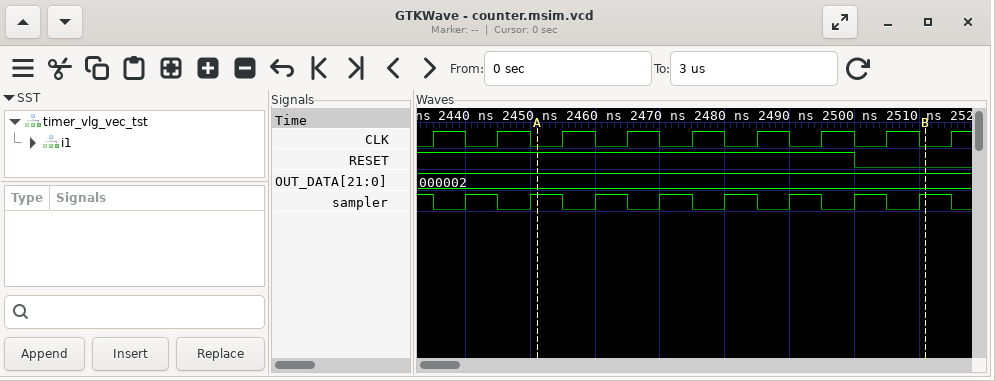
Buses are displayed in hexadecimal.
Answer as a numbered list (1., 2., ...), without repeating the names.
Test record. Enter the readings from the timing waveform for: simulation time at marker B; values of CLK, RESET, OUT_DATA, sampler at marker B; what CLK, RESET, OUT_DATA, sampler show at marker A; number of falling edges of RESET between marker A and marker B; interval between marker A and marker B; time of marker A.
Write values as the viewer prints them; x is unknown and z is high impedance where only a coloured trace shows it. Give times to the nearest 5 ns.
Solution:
1. 2510 ns
2. CLK=0, RESET=0, OUT_DATA=000002, sampler=1
3. CLK=0, RESET=1, OUT_DATA=000002, sampler=1
4. 1
5. 60 ns
6. 2450 ns
